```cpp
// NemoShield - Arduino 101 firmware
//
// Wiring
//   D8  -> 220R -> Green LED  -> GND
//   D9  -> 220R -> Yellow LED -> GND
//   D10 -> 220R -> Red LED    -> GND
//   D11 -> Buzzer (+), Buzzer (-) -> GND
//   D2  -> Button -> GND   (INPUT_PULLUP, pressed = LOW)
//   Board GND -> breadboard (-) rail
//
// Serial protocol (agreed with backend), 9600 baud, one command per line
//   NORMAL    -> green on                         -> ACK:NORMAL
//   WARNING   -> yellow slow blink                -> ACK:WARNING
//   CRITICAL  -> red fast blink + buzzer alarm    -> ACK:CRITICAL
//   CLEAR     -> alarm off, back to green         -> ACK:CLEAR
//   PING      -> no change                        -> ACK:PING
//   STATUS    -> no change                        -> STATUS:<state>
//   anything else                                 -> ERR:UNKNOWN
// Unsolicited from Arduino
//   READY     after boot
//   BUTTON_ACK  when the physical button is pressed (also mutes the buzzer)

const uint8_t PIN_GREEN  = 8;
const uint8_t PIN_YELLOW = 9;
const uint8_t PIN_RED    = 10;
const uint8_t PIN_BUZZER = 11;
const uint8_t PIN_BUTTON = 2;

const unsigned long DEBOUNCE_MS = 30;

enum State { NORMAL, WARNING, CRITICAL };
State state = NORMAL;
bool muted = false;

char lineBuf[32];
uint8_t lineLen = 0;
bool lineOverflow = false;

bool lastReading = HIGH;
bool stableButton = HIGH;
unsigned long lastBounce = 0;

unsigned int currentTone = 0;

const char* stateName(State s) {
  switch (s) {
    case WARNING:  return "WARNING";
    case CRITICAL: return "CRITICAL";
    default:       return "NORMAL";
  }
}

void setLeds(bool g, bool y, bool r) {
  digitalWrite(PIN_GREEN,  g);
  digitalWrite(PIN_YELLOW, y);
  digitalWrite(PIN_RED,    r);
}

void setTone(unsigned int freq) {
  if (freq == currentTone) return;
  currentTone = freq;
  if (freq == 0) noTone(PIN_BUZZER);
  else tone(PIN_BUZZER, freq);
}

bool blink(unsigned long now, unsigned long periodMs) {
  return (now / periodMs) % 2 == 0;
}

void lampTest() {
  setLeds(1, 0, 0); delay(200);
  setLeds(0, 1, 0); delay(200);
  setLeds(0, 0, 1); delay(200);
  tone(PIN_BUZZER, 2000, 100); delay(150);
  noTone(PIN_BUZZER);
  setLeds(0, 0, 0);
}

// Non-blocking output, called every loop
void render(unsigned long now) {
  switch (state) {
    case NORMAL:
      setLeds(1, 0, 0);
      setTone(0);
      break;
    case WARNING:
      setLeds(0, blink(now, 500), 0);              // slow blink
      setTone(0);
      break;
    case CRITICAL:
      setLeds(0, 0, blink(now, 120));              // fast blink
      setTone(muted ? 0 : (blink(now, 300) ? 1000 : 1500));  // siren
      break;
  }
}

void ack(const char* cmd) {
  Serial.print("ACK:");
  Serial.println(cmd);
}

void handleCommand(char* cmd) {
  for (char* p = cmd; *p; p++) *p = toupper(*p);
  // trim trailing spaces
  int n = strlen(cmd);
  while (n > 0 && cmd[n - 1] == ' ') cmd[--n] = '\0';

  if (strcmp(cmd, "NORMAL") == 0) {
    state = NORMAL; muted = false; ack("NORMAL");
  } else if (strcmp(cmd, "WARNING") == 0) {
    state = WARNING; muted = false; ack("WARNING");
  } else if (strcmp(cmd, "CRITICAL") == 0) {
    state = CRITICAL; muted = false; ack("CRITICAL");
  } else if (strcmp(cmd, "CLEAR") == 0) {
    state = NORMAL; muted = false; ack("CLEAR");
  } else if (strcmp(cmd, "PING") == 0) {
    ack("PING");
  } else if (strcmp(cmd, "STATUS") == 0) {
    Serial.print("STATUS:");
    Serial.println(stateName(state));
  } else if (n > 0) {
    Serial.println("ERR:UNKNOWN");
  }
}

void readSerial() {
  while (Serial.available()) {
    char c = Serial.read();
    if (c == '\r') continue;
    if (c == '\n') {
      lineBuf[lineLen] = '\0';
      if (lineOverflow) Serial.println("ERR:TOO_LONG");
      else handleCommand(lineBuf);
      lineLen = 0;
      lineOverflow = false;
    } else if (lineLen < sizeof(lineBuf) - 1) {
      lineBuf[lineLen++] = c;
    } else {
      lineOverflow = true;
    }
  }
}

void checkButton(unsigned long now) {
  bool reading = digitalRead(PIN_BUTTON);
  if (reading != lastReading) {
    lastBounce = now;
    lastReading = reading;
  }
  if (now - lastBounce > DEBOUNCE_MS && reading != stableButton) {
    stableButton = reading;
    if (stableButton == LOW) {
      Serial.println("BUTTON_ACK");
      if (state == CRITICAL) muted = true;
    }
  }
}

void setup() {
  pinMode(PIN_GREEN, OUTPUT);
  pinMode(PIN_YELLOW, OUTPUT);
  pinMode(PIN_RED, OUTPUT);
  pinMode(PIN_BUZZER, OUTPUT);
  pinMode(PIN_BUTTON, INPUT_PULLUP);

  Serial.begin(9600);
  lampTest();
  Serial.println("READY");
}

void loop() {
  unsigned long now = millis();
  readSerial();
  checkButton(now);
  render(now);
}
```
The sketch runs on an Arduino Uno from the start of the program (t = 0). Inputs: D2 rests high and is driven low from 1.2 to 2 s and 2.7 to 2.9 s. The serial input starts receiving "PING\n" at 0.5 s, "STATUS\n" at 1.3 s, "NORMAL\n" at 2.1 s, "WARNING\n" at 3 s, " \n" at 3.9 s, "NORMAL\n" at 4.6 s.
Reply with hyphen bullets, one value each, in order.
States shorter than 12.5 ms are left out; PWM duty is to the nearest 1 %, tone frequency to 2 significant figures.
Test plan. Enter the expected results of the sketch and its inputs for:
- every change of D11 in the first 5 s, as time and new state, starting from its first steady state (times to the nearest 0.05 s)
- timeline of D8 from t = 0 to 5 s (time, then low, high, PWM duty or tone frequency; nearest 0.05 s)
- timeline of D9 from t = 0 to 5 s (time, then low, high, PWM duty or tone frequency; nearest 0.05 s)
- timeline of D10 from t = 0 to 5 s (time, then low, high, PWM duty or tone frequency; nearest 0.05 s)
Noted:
- 0 s low; 0.6 s tone 2000 Hz; 0.7 s low
- 0 s high; 0.2 s low; 0.75 s high; 3 s low; 4.6 s high
- 0 s low; 0.2 s high; 0.4 s low; 3 s high; 3.5 s low; 4 s high; 4.5 s low
- 0 s low; 0.4 s high; 0.75 s low
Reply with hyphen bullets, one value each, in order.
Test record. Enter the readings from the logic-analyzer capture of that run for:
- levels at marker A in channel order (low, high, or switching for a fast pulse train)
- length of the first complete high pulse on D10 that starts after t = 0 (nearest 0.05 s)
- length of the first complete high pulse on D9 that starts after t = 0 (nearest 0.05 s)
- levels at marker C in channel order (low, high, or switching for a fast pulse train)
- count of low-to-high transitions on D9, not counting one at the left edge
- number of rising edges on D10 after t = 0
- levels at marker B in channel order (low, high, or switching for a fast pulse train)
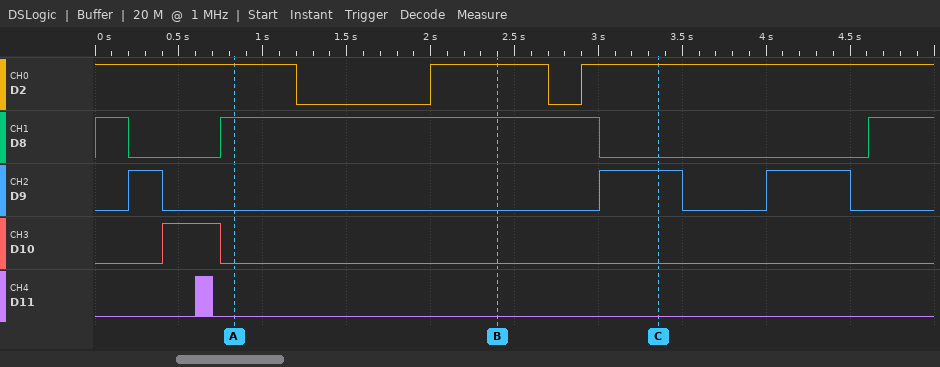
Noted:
- D2 high, D8 high, D9 low, D10 low, D11 low
- 0.35 s
- 0.20 s
- D2 high, D8 low, D9 high, D10 low, D11 low
- 3
- 1
- D2 high, D8 high, D9 low, D10 low, D11 low
